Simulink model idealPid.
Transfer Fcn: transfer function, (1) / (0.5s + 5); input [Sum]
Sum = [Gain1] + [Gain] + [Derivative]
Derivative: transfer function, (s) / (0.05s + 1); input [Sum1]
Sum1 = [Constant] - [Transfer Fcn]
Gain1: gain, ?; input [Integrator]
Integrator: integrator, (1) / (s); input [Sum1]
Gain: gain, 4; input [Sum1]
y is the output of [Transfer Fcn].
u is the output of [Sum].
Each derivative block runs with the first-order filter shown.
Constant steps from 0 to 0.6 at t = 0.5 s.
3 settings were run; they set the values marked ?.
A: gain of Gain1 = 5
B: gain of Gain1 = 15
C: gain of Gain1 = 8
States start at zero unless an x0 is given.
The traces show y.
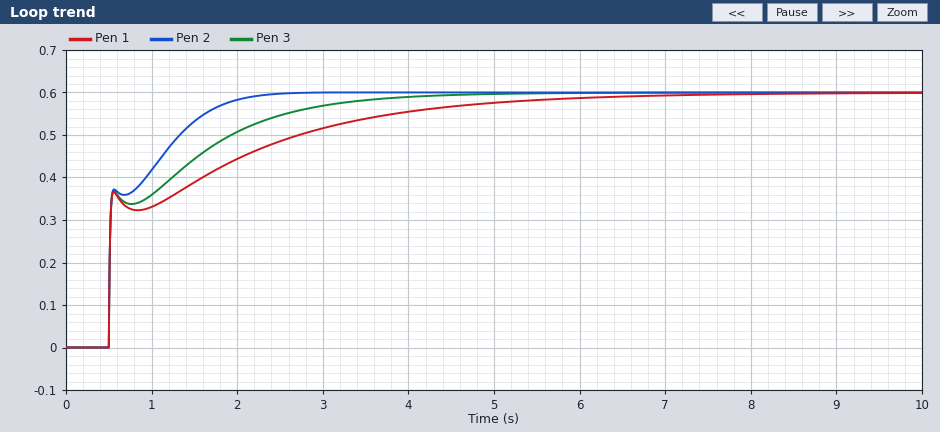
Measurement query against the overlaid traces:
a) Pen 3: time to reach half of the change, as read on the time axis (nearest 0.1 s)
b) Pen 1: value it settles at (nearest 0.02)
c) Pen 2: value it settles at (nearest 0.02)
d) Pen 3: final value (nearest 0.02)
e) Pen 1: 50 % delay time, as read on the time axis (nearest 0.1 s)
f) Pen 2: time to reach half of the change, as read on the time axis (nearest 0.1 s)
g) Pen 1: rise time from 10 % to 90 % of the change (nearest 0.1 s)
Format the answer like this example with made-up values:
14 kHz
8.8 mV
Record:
0.5 s
0.60
0.60
0.60
0.5 s
0.5 s
3.0 s
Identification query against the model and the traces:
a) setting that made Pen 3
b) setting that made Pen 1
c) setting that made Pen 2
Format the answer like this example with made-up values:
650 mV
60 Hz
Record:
C
A
B
